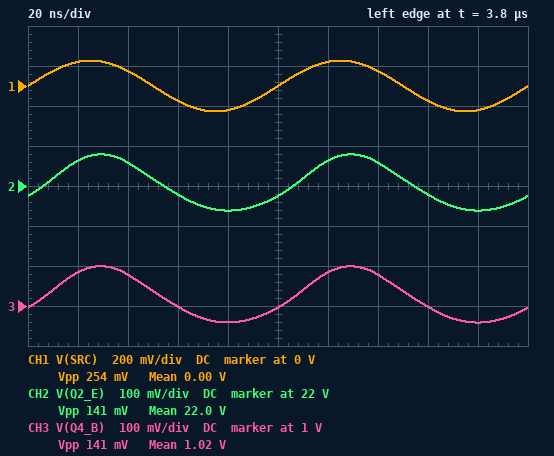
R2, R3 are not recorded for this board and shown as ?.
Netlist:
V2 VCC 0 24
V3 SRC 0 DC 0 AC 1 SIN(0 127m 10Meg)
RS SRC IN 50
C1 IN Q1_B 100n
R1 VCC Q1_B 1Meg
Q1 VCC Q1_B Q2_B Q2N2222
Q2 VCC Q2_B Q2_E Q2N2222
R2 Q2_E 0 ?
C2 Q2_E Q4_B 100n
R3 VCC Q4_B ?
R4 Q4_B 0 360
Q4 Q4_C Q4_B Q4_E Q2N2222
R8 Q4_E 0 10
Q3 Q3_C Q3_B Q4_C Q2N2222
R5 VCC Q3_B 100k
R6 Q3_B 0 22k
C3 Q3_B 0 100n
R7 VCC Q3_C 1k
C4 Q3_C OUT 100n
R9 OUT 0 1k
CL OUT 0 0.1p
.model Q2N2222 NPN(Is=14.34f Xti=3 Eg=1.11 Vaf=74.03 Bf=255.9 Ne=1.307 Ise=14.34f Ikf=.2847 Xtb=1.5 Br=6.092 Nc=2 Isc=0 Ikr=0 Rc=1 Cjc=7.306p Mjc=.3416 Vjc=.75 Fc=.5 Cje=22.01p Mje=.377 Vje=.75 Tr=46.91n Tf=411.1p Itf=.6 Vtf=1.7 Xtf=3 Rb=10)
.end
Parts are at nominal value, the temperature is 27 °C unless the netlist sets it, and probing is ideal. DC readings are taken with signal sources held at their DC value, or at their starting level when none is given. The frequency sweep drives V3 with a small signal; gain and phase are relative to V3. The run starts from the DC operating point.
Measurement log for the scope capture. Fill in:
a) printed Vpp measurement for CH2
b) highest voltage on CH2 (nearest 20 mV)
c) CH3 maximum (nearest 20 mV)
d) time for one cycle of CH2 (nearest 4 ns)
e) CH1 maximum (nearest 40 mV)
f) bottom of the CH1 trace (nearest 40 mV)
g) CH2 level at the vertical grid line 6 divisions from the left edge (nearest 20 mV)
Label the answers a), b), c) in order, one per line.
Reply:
a) 141 mV
b) 22.08 V
c) 1.10 V
d) 100 ns
e) 120 mV
f) -120 mV
g) 22.06 V
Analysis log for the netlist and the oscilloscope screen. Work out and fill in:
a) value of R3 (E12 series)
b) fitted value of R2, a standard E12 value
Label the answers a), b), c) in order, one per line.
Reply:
a) 4.7 kΩ
b) 1.5 kΩ
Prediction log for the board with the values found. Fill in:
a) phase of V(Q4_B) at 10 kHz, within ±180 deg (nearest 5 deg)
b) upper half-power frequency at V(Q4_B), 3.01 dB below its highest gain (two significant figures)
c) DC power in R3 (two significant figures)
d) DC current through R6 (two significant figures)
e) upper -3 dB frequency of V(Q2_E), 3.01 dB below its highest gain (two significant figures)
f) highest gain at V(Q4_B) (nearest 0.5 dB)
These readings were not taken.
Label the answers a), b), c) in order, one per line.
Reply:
a) 80 deg
b) 13 MHz
c) 110 mW
d) 48 µA
e) 6.2 MHz
f) -1.5 dB
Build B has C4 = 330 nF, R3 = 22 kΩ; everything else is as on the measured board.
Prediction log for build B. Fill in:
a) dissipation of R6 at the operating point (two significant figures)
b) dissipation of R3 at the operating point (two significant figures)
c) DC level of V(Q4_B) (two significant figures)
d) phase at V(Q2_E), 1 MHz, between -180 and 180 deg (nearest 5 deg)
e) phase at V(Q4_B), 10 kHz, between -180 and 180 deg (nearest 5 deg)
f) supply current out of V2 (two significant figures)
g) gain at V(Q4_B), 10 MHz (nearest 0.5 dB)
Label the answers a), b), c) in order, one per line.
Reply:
a) 850 µW
b) 25 mW
c) 390 mV
d) 0 deg
e) 25 deg
f) 16 mA
g) -0.5 dB
